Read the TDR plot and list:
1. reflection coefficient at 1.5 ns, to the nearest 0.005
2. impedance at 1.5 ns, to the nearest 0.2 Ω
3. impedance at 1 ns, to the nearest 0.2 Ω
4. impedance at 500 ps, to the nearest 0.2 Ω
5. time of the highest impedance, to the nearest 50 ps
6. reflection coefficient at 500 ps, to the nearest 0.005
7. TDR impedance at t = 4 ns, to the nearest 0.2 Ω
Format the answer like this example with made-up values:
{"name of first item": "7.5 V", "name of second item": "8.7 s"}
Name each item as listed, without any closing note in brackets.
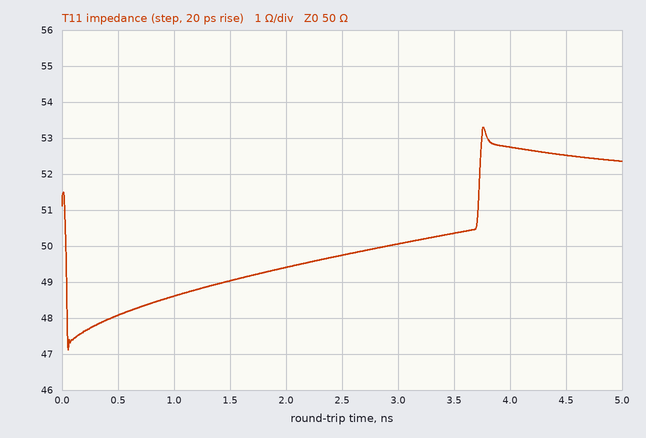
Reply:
{"reflection coefficient at 1.5 ns, to the nearest 0.005": "-0.010", "impedance at 1.5 ns, to the nearest 0.2 Ω": "49.0 Ω", "impedance at 1 ns, to the nearest 0.2 Ω": "48.6 Ω", "impedance at 500 ps, to the nearest 0.2 Ω": "48.0 Ω", "time of the highest impedance, to the nearest 50 ps": "3.75 ns", "reflection coefficient at 500 ps, to the nearest 0.005": "-0.020", "TDR impedance at t = 4 ns, to the nearest 0.2 Ω": "52.8 Ω"}
